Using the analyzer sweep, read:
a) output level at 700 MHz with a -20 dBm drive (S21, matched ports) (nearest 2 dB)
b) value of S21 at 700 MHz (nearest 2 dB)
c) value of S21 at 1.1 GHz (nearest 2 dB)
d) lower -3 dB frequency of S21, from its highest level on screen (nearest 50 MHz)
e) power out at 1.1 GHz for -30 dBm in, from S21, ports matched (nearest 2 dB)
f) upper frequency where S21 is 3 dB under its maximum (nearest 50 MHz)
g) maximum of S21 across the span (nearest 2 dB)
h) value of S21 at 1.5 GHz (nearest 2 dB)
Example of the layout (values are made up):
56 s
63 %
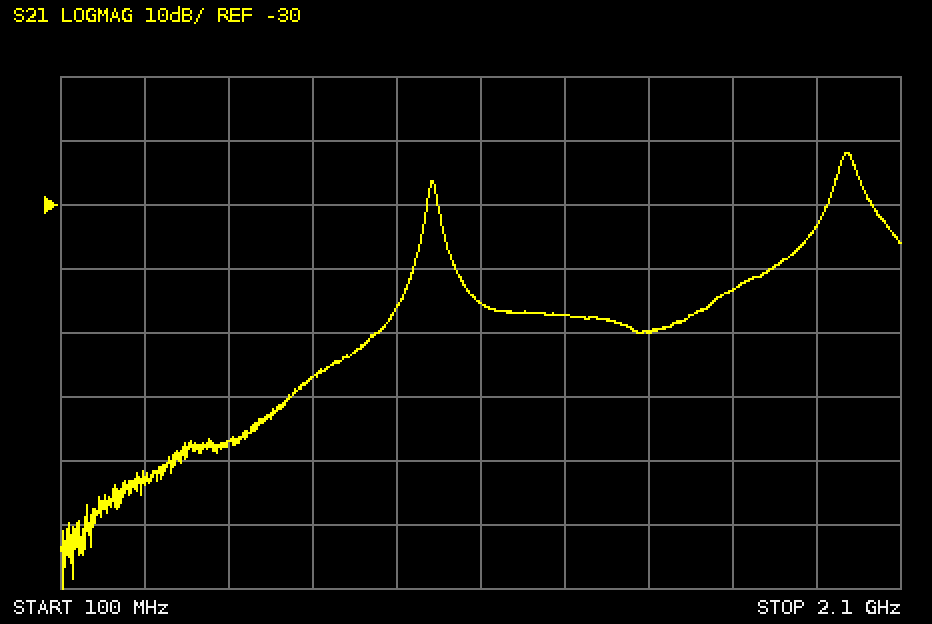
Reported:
-76 dBm
-56 dB
-46 dB
1.95 GHz
-76 dBm
2.00 GHz
-22 dB
-50 dB
